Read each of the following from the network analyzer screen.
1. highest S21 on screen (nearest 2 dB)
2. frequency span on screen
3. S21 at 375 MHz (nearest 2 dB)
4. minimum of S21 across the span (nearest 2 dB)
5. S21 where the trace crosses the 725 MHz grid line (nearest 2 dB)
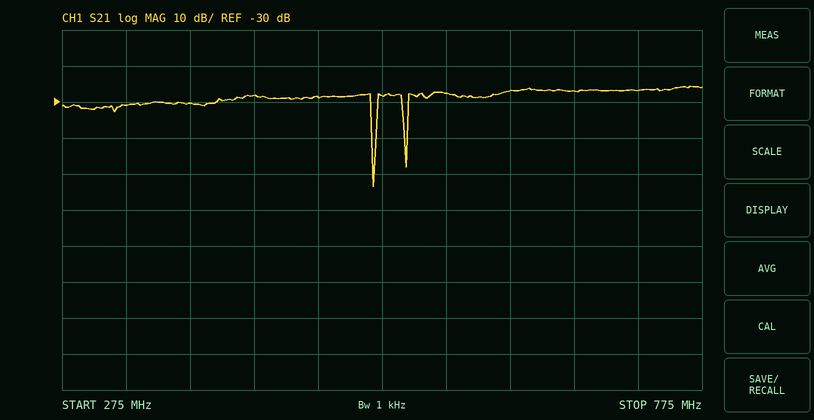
-26 dB
500 MHz
-30 dB
-54 dB
-26 dB
